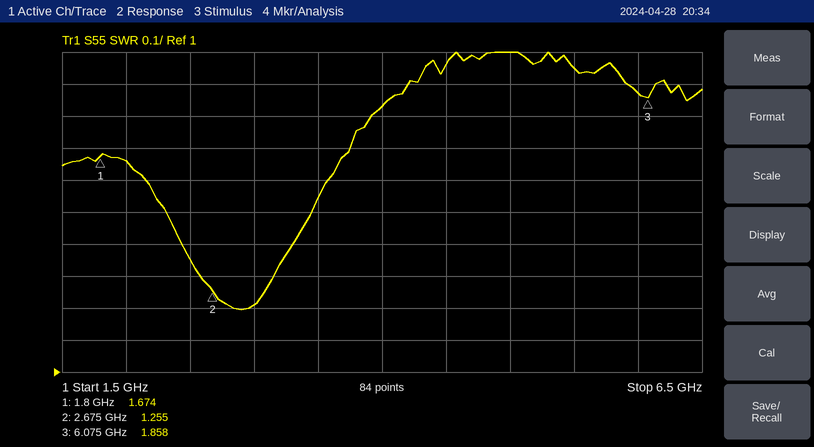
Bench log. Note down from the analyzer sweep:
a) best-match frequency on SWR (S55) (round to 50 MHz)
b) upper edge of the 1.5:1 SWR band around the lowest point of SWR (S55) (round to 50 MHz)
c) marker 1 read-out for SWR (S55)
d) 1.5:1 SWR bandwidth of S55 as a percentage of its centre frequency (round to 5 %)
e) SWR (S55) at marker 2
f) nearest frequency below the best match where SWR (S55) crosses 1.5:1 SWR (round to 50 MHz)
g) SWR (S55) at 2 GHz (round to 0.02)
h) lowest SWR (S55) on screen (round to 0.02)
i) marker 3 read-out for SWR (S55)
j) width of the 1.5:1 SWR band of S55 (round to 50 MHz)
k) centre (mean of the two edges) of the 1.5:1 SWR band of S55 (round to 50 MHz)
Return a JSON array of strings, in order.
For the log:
["2.90 GHz", "3.45 GHz", "1.674", "40 %", "1.255", "2.30 GHz", "1.66", "1.20", "1.858", "1.15 GHz", "2.90 GHz"]
